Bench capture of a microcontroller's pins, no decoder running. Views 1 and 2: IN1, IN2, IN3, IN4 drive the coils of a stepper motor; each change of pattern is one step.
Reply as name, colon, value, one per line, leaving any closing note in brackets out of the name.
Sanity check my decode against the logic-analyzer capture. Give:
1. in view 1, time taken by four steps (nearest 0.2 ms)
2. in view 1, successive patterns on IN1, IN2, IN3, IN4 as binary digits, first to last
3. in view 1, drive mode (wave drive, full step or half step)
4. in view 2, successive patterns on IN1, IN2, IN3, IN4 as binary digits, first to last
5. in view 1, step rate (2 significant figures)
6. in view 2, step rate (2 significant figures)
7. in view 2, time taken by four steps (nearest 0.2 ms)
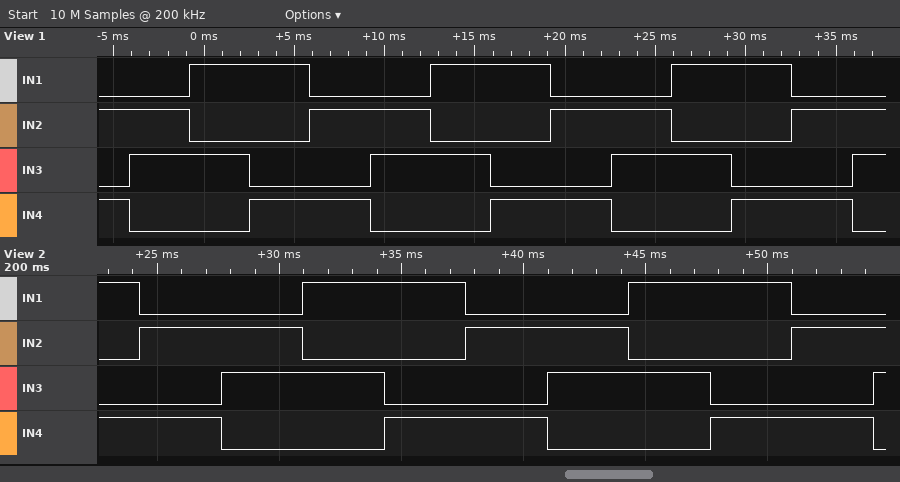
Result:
in view 1, time taken by four steps: 13.4 ms
in view 1, successive patterns on IN1, IN2, IN3, IN4 as binary digits, first to last: 0101 0110 1010 1001 0101 0110 1010 1001 0101 0110 1010 1001 0101 0110
in view 1, drive mode: full step
in view 2, successive patterns on IN1, IN2, IN3, IN4 as binary digits, first to last: 1001 0101 0110 1010 1001 0101 0110 1010 1001 0101 0110
in view 1, step rate: 300 steps/s
in view 2, step rate: 300 steps/s
in view 2, time taken by four steps: 13.4 ms
